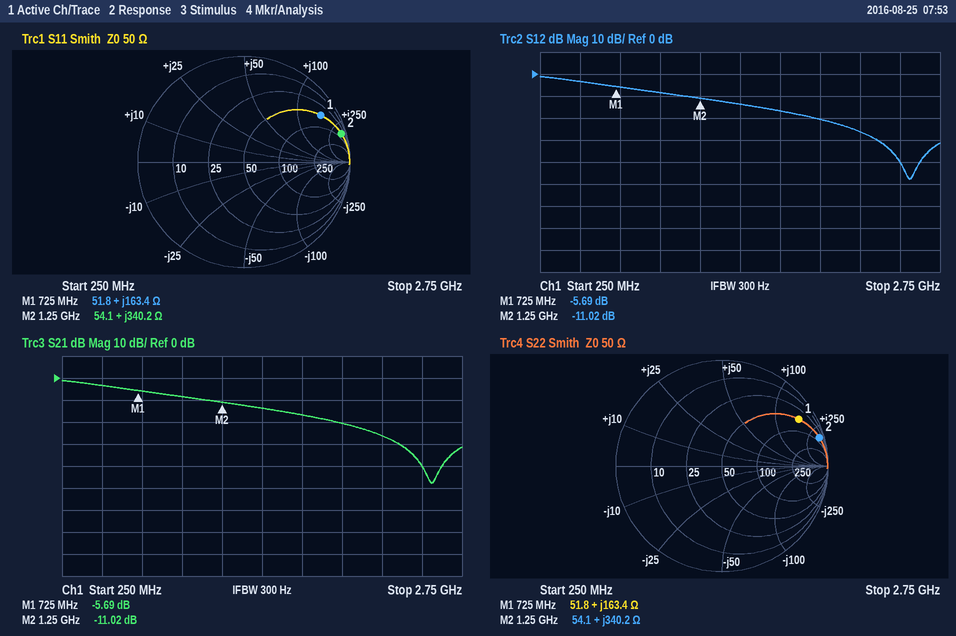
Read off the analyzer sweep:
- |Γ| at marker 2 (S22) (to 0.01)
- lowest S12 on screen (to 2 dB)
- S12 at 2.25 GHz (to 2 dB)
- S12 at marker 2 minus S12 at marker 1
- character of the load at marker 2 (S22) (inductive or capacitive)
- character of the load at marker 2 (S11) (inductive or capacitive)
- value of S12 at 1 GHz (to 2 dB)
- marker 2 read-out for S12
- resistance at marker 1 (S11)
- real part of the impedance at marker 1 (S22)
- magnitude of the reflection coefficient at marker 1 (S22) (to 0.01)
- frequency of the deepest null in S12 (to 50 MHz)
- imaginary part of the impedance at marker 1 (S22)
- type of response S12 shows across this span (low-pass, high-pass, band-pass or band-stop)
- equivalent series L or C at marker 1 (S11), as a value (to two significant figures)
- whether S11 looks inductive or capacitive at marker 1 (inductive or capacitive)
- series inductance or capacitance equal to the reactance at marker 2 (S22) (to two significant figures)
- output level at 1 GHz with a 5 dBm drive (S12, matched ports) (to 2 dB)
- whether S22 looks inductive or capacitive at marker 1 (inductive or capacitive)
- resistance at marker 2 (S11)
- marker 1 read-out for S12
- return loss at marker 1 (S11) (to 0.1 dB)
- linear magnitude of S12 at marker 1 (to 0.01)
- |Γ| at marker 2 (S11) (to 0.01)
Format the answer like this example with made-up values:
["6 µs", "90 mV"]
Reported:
["0.96", "-48 dB", "-26 dB", "-5.33 dB", "inductive", "inductive", "-8 dB", "-11.02 dB", "51.8 Ω", "51.8 Ω", "0.85", "2.55 GHz", "+163.4 Ω", "low-pass", "36 nH", "inductive", "43 nH", "-4 dBm", "inductive", "54.1 Ω", "-5.69 dB", "1.4 dB", "0.52", "0.96"]
